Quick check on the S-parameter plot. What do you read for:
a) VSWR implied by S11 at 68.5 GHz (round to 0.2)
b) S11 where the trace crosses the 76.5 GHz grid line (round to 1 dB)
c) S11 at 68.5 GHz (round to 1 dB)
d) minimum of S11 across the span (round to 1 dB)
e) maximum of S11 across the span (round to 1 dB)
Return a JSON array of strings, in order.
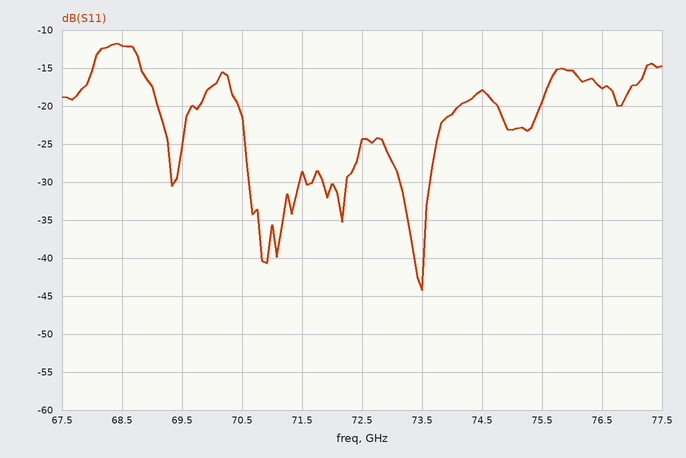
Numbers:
["1.6", "-18 dB", "-12 dB", "-44 dB", "-12 dB"]
